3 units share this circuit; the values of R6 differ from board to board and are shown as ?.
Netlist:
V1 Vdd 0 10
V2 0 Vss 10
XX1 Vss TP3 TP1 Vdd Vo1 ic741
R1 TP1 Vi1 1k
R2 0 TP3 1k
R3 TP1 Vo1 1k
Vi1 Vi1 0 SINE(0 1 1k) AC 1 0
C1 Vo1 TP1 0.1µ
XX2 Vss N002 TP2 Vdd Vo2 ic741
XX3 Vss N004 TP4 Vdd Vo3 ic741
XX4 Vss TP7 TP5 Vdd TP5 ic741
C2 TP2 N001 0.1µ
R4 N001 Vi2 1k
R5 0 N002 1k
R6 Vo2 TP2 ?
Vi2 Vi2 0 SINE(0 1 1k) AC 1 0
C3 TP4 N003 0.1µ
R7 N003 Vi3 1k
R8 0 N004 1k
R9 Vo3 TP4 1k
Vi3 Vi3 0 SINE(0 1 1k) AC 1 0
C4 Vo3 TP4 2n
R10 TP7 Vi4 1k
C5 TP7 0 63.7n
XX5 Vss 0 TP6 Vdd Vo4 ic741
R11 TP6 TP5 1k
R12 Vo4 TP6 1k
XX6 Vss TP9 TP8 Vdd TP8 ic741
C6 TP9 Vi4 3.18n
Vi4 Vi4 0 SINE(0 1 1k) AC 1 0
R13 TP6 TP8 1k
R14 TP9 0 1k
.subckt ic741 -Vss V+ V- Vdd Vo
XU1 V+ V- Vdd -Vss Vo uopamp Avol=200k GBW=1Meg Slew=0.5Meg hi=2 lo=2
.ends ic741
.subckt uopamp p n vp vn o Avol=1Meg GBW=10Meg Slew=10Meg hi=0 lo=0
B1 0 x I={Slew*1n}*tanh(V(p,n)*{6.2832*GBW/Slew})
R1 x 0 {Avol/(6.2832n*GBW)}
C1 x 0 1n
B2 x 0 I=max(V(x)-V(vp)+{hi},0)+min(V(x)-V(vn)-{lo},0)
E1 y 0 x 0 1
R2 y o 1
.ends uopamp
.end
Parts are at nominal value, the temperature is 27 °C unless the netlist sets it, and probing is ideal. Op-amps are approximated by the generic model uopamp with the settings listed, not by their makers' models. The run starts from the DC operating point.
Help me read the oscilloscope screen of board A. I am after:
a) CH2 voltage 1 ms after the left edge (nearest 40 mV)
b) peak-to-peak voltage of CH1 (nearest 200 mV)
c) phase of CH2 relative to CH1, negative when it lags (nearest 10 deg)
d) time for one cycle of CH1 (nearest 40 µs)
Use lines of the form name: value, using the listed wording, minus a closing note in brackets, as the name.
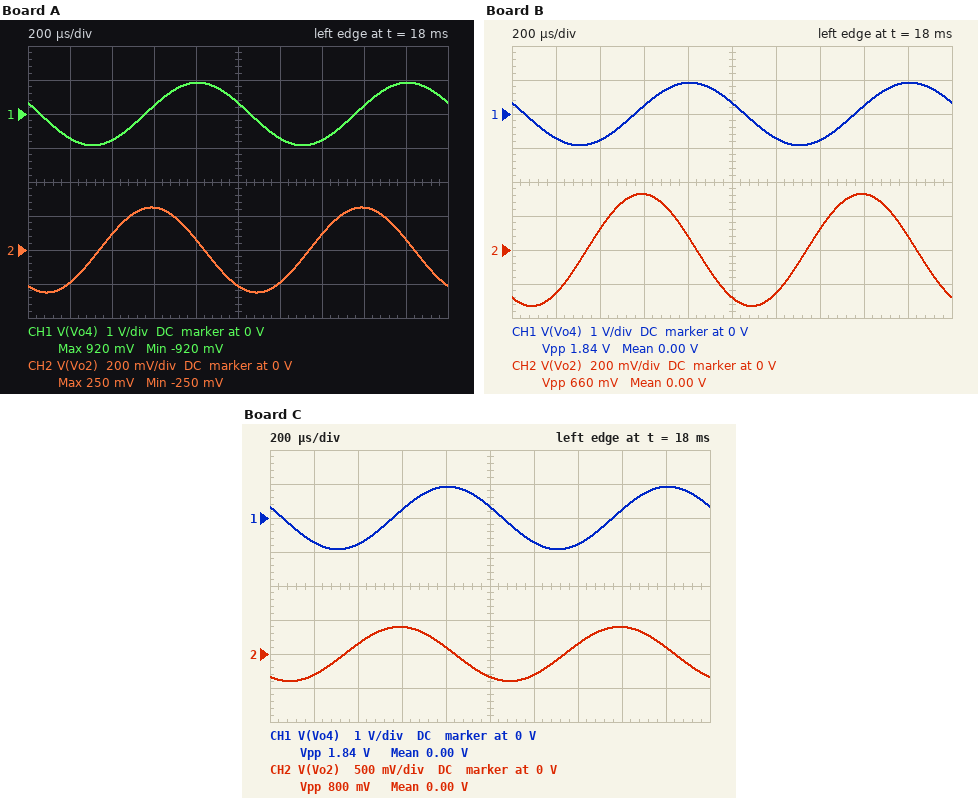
CH2 voltage 1 ms after the left edge: -200 mV
peak-to-peak voltage of CH1: 1.8 V
phase of CH2 relative to CH1, negative when it lags: 80 deg
time for one cycle of CH1: 1.00 ms
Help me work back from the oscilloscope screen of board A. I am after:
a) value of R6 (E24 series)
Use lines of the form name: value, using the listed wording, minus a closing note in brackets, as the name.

value of R6: 470 Ω
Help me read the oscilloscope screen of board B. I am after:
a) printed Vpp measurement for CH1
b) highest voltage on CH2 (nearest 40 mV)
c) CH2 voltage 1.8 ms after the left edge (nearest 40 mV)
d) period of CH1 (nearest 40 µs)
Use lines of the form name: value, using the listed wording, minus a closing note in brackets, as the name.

printed Vpp measurement for CH1: 1.84 V
highest voltage on CH2: 320 mV
CH2 voltage 1.8 ms after the left edge: 80 mV
period of CH1: 1.00 ms
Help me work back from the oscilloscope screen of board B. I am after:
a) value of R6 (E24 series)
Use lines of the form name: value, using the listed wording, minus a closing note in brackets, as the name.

value of R6: 620 Ω
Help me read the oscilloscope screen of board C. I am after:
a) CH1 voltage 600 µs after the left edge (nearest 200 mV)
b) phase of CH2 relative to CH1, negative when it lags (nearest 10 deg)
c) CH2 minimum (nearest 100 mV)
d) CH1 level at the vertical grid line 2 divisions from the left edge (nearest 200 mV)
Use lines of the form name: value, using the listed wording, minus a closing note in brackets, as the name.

CH1 voltage 600 µs after the left edge: 200 mV
phase of CH2 relative to CH1, negative when it lags: 80 deg
CH2 minimum: -400 mV
CH1 level at the vertical grid line 2 divisions from the left edge: -800 mV
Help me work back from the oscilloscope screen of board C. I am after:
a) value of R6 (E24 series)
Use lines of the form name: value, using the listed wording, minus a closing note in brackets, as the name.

value of R6: 750 Ω
